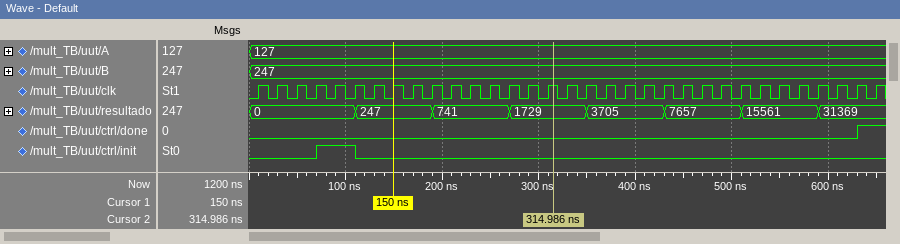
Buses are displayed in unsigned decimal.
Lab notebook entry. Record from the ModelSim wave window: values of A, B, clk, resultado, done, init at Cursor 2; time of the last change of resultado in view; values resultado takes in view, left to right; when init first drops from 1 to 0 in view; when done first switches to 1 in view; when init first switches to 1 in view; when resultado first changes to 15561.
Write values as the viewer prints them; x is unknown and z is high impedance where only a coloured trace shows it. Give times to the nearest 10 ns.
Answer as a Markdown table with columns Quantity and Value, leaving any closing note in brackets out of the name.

| Quantity | Value |
|---|---|
| values of A, B, clk, resultado, done, init at Cursor 2 | A=127, B=247, clk=1, resultado=1729, done=0, init=0 |
| time of the last change of resultado in view | 590 ns |
| values resultado takes in view, left to right | 0, 247, 741, 1729, 3705, 7657, 15561, 31369 |
| when init first drops from 1 to 0 in view | 110 ns |
| when done first switches to 1 in view | 630 ns |
| when init first switches to 1 in view | 70 ns |
| when resultado first changes to 15561 | 510 ns |
